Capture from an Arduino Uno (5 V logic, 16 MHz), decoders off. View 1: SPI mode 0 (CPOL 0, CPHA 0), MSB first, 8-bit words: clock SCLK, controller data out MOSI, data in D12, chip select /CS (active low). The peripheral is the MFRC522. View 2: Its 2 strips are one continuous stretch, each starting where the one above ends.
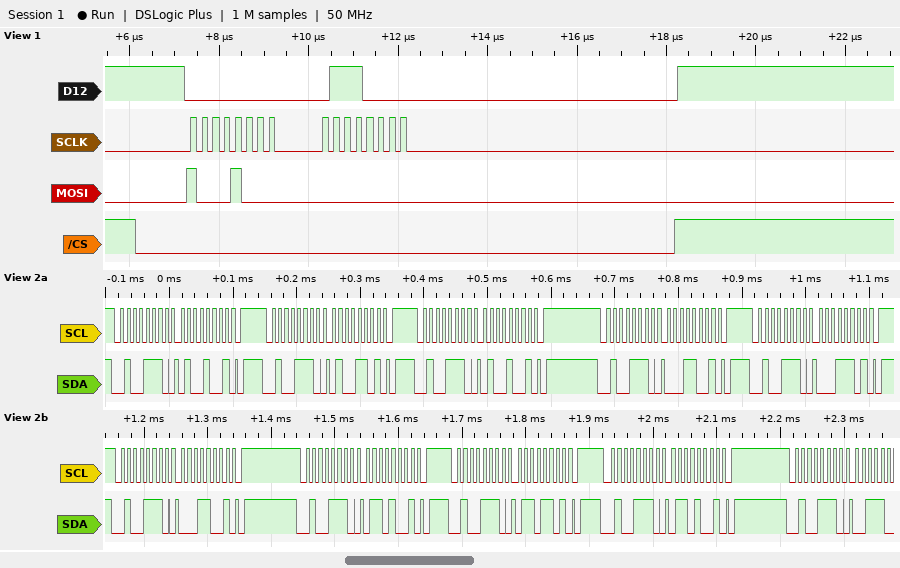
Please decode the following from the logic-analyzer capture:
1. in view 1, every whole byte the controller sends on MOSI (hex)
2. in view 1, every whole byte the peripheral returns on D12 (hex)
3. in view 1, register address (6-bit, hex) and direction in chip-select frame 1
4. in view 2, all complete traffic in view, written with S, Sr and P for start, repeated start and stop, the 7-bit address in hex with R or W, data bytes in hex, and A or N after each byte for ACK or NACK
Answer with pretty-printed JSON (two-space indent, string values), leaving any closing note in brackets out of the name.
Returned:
{
  "in view 1, every whole byte the controller sends on MOSI": "88 00",
  "in view 1, every whole byte the peripheral returns on D12": "00 70",
  "in view 1, register address (6-bit, hex) and direction in chip-select frame 1": "0x04 read",
  "in view 2, all complete traffic in view, written with S, Sr and P for start, repeated start and stop, the 7-bit address in hex with R or W, data bytes in hex, and A or N after each byte for ACK or NACK": "S 27W A 49 A P S 27W A 4D A P S 27W A 49 A P S 27W A 19 A P S 27W A 1D A P S 27W A 19 A P S 27W A 69 A P S 27W A 6D A P S 27W A 69 A P S 27W A"
}
